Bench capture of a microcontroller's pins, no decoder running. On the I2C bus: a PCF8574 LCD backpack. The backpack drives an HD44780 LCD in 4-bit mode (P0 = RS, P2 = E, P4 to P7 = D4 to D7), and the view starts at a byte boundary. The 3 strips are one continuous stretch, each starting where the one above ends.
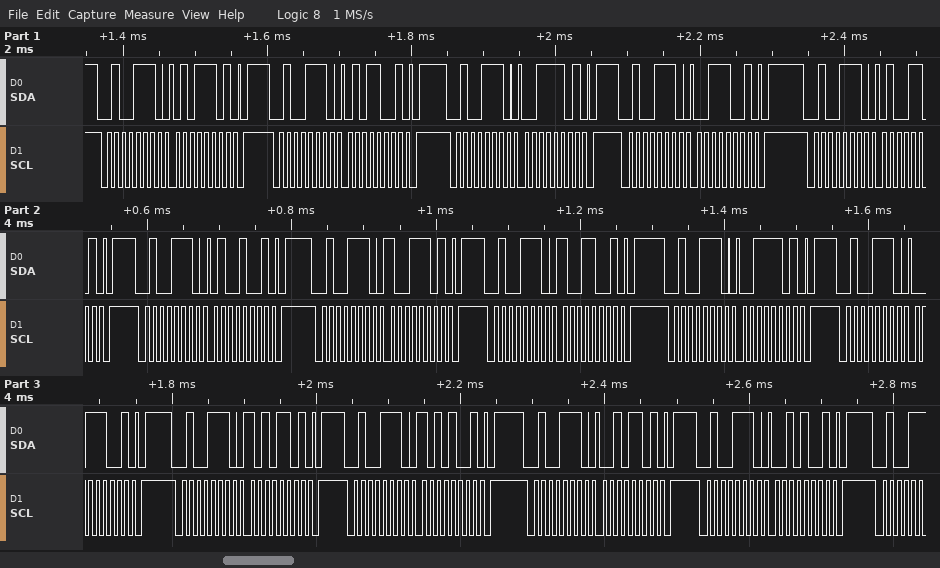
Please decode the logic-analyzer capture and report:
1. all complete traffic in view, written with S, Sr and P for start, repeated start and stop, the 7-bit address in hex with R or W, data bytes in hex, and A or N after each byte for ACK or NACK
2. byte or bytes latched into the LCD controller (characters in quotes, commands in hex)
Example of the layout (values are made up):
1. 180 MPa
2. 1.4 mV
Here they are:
1. S 27W A 5D A P S 27W A 59 A P S 27W A 3D A P S 27W A 39 A P S 27W A 4D A P S 27W A 49 A P S 27W A 9D A P S 27W A 99 A P S 27W A 3D A P S 27W A 39 A P S 27W A AD A P S 27W A A9 A P S 27W A 2D A P S 27W A 29 A P
2. 'S' 'I' ':'
